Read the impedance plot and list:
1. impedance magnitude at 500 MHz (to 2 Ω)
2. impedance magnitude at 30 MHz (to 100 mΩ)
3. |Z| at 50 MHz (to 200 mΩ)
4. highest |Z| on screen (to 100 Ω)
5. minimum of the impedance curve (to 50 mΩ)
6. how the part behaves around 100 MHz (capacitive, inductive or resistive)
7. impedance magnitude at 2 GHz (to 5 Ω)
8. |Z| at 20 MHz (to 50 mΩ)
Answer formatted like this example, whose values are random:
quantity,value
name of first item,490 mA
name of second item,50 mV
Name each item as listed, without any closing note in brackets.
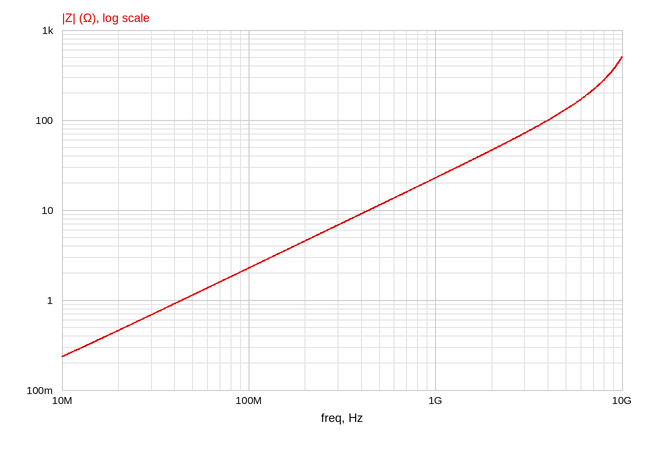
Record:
quantity,value
impedance magnitude at 500 MHz,12 Ω
impedance magnitude at 30 MHz,700 mΩ
|Z| at 50 MHz,1.2 Ω
highest |Z| on screen,500 Ω
minimum of the impedance curve,250 mΩ
how the part behaves around 100 MHz,inductive
impedance magnitude at 2 GHz,45 Ω
|Z| at 20 MHz,450 mΩ
